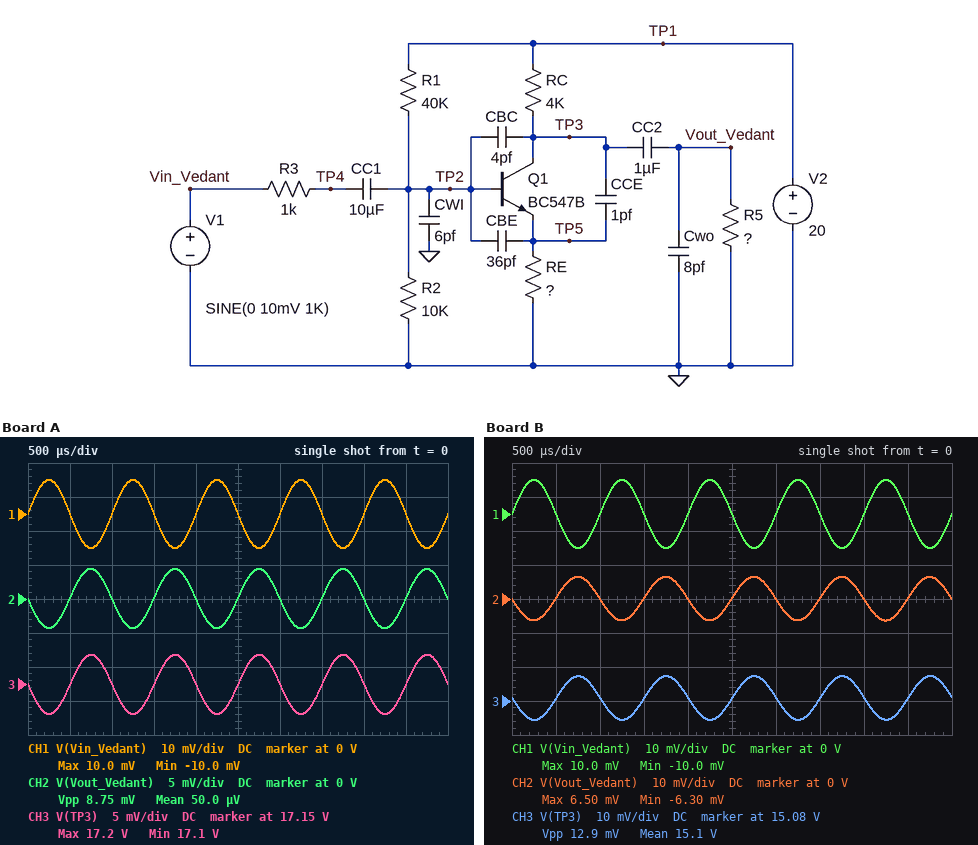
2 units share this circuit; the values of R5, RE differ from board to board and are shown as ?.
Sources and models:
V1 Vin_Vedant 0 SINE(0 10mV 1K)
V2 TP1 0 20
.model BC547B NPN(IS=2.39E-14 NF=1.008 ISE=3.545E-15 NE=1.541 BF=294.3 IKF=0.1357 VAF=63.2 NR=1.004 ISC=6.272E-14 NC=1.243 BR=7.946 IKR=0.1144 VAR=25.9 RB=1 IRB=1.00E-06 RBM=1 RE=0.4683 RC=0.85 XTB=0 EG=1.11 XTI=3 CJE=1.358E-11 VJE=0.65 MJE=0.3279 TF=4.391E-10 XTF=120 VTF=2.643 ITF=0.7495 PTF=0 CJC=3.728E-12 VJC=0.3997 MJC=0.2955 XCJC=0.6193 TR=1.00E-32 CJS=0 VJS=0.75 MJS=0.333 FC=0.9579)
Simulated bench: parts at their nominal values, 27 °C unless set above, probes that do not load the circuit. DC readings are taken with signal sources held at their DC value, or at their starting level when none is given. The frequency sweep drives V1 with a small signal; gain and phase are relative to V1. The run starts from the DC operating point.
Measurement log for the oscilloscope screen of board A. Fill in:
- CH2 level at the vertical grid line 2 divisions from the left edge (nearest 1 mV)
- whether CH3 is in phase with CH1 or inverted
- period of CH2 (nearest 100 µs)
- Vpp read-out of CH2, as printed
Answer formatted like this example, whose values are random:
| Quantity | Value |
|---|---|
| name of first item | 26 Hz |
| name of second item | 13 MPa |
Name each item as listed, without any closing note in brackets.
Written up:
| Quantity | Value |
|---|---|
| CH2 level at the vertical grid line 2 divisions from the left edge | 0 V |
| whether CH3 is in phase with CH1 or inverted | inverted |
| period of CH2 | 1.0 ms |
| Vpp read-out of CH2, as printed | 8.75 mV |
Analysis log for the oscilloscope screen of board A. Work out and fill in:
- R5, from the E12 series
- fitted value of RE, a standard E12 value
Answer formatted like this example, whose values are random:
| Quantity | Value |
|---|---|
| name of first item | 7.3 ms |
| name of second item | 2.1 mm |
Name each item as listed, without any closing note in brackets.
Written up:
| Quantity | Value |
|---|---|
| R5, from the E12 series | 5.6 kΩ |
| fitted value of RE, a standard E12 value | 4.7 kΩ |
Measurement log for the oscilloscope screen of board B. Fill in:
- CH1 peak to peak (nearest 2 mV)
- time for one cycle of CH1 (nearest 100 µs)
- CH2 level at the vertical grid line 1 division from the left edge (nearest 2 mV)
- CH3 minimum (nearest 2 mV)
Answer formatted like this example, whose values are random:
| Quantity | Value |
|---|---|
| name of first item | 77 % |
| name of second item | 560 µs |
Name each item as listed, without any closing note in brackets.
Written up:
| Quantity | Value |
|---|---|
| CH1 peak to peak | 20 mV |
| time for one cycle of CH1 | 1.0 ms |
| CH2 level at the vertical grid line 1 division from the left edge | 0 V |
| CH3 minimum | 15.074 V |
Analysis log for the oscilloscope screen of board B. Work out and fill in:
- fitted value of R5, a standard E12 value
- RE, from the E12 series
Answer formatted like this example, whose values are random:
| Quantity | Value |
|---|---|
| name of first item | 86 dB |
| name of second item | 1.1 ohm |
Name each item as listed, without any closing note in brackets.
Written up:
| Quantity | Value |
|---|---|
| fitted value of R5, a standard E12 value | 3.9 kΩ |
| RE, from the E12 series | 2.7 kΩ |
